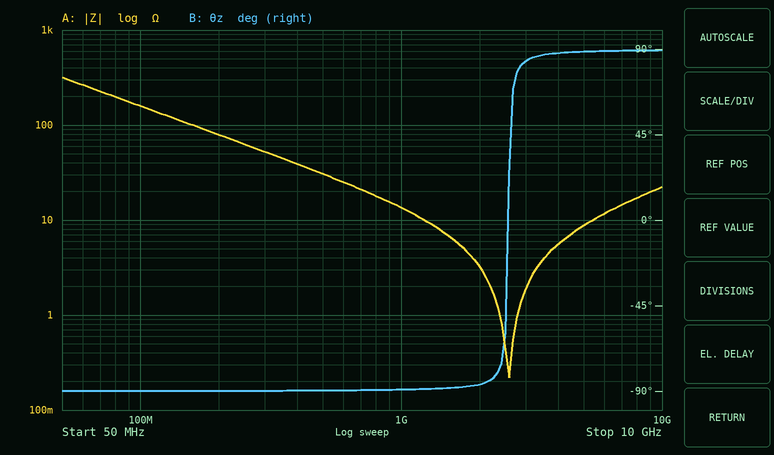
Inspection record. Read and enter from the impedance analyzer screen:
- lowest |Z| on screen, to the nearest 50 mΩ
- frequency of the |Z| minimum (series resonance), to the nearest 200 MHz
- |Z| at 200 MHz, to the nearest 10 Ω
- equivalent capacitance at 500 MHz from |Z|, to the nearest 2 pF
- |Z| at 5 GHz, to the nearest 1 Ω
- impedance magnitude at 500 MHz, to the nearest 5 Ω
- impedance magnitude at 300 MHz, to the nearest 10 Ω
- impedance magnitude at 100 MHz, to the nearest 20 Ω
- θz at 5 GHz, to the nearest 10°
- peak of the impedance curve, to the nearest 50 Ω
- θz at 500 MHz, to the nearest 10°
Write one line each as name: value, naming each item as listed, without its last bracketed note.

lowest |Z| on screen, to the nearest 50 mΩ: 200 mΩ
frequency of the |Z| minimum (series resonance), to the nearest 200 MHz: 2.6 GHz
|Z| at 200 MHz, to the nearest 10 Ω: 80 Ω
equivalent capacitance at 500 MHz from |Z|, to the nearest 2 pF: 10 pF
|Z| at 5 GHz, to the nearest 1 Ω: 9 Ω
impedance magnitude at 500 MHz, to the nearest 5 Ω: 30 Ω
impedance magnitude at 300 MHz, to the nearest 10 Ω: 50 Ω
impedance magnitude at 100 MHz, to the nearest 20 Ω: 160 Ω
θz at 5 GHz, to the nearest 10°: 90°
peak of the impedance curve, to the nearest 50 Ω: 300 Ω
θz at 500 MHz, to the nearest 10°: -90°
